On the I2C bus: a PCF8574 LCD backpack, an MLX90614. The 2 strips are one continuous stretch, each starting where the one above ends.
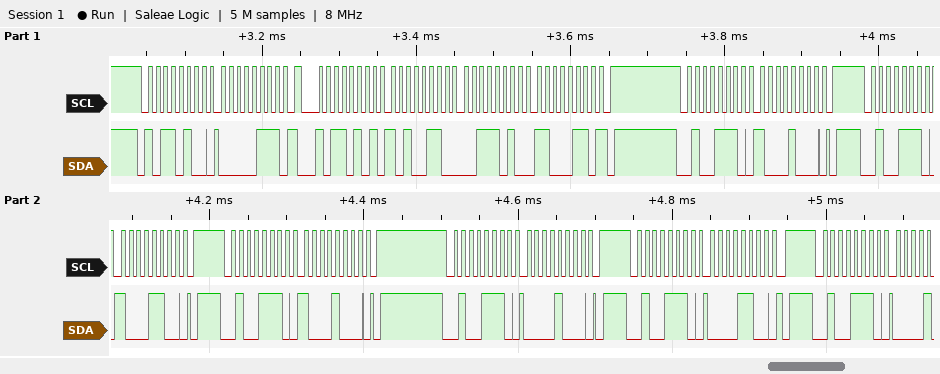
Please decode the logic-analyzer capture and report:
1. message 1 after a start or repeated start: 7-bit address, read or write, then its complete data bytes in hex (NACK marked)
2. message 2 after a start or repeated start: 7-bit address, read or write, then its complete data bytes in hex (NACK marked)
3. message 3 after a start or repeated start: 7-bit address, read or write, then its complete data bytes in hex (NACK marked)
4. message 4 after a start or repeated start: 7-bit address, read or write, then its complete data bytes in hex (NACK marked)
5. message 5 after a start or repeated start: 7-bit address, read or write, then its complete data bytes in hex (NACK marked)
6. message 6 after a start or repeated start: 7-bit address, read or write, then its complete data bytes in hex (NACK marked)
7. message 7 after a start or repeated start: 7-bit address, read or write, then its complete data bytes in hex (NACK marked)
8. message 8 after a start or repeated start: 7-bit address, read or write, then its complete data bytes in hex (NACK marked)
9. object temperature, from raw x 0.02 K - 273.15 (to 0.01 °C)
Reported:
0x5A write: 07
0x5A read: A6 3A C6 NACK
0x27 write: 88
0x27 write: 8C
0x27 write: 88
0x27 write: 08
0x27 write: 0C
0x27 write
27.13 °C
